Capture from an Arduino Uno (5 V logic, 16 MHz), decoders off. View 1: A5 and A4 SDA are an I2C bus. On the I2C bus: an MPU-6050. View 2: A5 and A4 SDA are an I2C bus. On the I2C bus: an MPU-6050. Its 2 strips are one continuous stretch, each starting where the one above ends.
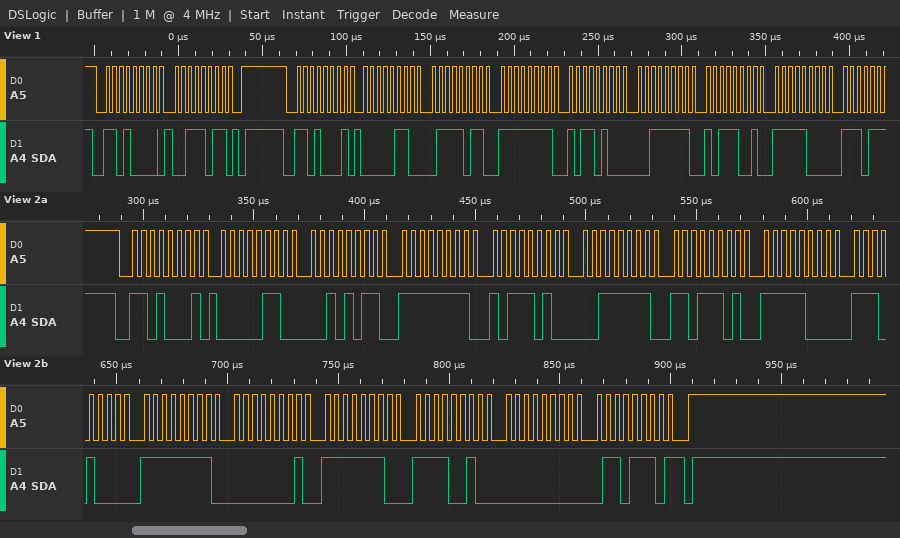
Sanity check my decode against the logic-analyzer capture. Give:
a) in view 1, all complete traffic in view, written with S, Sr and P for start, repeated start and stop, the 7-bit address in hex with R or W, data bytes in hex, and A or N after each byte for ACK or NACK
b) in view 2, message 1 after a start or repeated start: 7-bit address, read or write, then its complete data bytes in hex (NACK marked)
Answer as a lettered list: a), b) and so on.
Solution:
a) S 68W A 3B A P S 68R A 06 A 7B A FF A B4 A 3F A B9 A F8 A
b) 0x68 read: 06 2B FF BA 3F DD F8 E8 FF 01 FE F2 00 6E NACK
